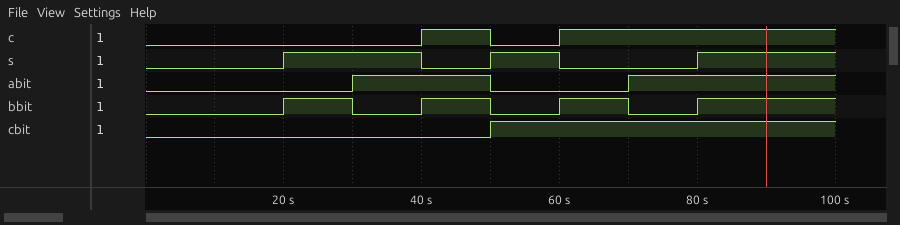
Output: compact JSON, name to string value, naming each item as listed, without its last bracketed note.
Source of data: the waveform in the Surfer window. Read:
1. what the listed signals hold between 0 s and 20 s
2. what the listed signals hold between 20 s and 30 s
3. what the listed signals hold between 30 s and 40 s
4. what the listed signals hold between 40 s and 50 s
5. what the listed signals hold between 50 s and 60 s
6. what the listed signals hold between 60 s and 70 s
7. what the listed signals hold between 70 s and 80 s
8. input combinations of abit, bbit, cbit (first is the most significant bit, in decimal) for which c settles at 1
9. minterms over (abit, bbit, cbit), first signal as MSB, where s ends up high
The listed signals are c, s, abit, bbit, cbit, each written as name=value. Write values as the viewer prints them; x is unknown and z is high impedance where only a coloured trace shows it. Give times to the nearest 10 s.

{"what the listed signals hold between 0 s and 20 s": "c=0, s=0, abit=0, bbit=0, cbit=0", "what the listed signals hold between 20 s and 30 s": "c=0, s=1, abit=0, bbit=1, cbit=0", "what the listed signals hold between 30 s and 40 s": "c=0, s=1, abit=1, bbit=0, cbit=0", "what the listed signals hold between 40 s and 50 s": "c=1, s=0, abit=1, bbit=1, cbit=0", "what the listed signals hold between 50 s and 60 s": "c=0, s=1, abit=0, bbit=0, cbit=1", "what the listed signals hold between 60 s and 70 s": "c=1, s=0, abit=0, bbit=1, cbit=1", "what the listed signals hold between 70 s and 80 s": "c=1, s=0, abit=1, bbit=0, cbit=1", "input combinations of abit, bbit, cbit (first is the most significant bit, in decimal) for which c settles at 1": "3, 5, 6, 7", "minterms over (abit, bbit, cbit), first signal as MSB, where s ends up high": "1, 2, 4, 7"}
